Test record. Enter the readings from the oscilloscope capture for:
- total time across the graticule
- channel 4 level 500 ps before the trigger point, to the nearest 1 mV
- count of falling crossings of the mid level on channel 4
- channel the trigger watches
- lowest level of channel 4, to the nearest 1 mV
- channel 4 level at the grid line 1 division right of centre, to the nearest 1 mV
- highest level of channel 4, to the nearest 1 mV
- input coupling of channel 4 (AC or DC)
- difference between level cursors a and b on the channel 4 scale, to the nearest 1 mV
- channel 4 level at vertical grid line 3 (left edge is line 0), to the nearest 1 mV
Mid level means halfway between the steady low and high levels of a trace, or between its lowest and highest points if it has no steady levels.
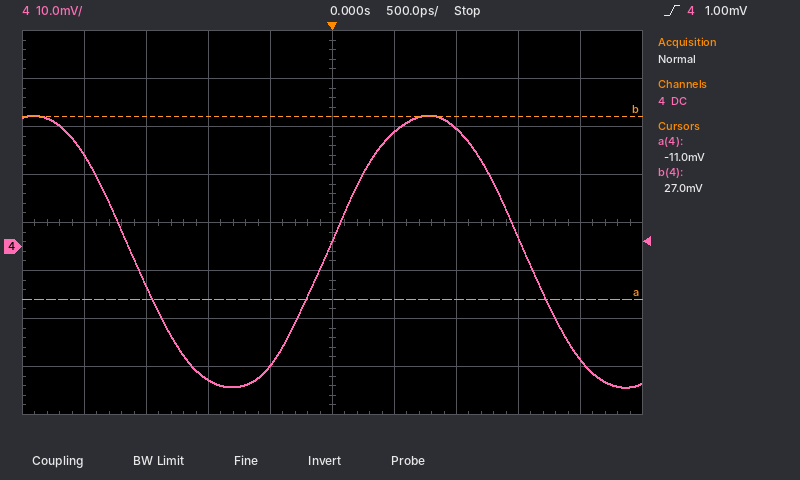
5 ns
-25 mV
2
channel 4
-29 mV
24 mV
27 mV
DC
38 mV
-28 mV
